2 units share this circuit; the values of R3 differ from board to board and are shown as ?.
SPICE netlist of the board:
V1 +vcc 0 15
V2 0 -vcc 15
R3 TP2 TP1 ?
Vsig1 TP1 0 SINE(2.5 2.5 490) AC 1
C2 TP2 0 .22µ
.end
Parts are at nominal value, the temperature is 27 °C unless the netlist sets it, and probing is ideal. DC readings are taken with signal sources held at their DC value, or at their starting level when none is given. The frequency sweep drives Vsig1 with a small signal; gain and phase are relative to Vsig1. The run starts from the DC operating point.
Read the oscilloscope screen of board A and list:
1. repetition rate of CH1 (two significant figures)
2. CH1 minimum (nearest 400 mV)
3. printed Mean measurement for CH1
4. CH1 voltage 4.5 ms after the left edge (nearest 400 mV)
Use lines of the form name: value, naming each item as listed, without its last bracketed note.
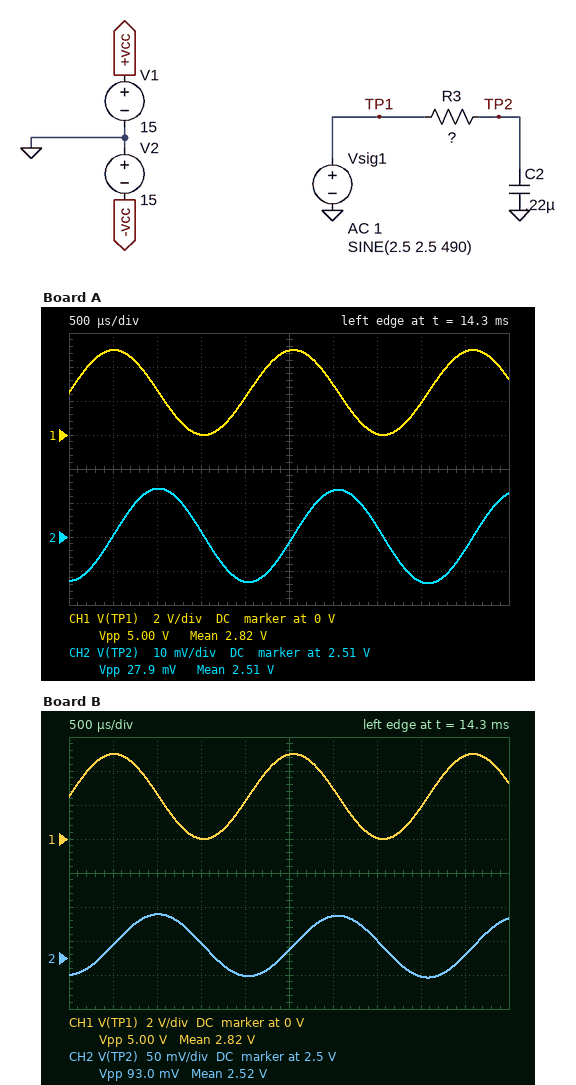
repetition rate of CH1: 490 Hz
CH1 minimum: 0 V
printed Mean measurement for CH1: 2.82 V
CH1 voltage 4.5 ms after the left edge: 4.8 V
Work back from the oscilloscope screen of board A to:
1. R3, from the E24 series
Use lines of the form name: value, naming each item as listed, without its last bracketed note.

R3, from the E24 series: 270 kΩ
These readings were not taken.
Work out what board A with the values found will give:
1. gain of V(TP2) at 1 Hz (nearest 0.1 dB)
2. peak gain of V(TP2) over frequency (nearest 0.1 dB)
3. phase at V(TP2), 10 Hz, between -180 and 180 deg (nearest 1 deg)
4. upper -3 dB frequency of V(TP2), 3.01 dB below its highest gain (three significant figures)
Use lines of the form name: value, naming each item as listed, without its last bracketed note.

gain of V(TP2) at 1 Hz: -0.6 dB
peak gain of V(TP2) over frequency: 0 dB
phase at V(TP2), 10 Hz, between -180 and 180 deg: -75 deg
upper -3 dB frequency of V(TP2), 3.01 dB below its highest gain: 2.68 Hz
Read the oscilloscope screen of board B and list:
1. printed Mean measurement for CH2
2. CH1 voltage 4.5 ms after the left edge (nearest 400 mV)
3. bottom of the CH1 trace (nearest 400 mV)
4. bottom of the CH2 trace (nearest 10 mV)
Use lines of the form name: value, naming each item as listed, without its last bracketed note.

printed Mean measurement for CH2: 2.52 V
CH1 voltage 4.5 ms after the left edge: 4.8 V
bottom of the CH1 trace: 0 V
bottom of the CH2 trace: 2.47 V
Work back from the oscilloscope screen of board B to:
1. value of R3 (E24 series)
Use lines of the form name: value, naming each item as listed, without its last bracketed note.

value of R3: 82 kΩ
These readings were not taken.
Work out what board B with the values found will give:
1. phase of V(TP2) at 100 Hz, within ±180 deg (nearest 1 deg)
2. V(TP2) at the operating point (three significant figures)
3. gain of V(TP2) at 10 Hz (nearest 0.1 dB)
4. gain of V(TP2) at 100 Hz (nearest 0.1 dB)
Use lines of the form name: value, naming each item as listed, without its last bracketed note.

phase of V(TP2) at 100 Hz, within ±180 deg: -85 deg
V(TP2) at the operating point: 2.50 V
gain of V(TP2) at 10 Hz: -3.6 dB
gain of V(TP2) at 100 Hz: -21.1 dB
